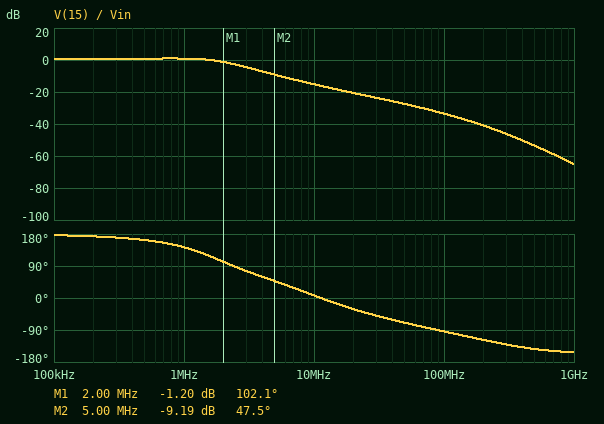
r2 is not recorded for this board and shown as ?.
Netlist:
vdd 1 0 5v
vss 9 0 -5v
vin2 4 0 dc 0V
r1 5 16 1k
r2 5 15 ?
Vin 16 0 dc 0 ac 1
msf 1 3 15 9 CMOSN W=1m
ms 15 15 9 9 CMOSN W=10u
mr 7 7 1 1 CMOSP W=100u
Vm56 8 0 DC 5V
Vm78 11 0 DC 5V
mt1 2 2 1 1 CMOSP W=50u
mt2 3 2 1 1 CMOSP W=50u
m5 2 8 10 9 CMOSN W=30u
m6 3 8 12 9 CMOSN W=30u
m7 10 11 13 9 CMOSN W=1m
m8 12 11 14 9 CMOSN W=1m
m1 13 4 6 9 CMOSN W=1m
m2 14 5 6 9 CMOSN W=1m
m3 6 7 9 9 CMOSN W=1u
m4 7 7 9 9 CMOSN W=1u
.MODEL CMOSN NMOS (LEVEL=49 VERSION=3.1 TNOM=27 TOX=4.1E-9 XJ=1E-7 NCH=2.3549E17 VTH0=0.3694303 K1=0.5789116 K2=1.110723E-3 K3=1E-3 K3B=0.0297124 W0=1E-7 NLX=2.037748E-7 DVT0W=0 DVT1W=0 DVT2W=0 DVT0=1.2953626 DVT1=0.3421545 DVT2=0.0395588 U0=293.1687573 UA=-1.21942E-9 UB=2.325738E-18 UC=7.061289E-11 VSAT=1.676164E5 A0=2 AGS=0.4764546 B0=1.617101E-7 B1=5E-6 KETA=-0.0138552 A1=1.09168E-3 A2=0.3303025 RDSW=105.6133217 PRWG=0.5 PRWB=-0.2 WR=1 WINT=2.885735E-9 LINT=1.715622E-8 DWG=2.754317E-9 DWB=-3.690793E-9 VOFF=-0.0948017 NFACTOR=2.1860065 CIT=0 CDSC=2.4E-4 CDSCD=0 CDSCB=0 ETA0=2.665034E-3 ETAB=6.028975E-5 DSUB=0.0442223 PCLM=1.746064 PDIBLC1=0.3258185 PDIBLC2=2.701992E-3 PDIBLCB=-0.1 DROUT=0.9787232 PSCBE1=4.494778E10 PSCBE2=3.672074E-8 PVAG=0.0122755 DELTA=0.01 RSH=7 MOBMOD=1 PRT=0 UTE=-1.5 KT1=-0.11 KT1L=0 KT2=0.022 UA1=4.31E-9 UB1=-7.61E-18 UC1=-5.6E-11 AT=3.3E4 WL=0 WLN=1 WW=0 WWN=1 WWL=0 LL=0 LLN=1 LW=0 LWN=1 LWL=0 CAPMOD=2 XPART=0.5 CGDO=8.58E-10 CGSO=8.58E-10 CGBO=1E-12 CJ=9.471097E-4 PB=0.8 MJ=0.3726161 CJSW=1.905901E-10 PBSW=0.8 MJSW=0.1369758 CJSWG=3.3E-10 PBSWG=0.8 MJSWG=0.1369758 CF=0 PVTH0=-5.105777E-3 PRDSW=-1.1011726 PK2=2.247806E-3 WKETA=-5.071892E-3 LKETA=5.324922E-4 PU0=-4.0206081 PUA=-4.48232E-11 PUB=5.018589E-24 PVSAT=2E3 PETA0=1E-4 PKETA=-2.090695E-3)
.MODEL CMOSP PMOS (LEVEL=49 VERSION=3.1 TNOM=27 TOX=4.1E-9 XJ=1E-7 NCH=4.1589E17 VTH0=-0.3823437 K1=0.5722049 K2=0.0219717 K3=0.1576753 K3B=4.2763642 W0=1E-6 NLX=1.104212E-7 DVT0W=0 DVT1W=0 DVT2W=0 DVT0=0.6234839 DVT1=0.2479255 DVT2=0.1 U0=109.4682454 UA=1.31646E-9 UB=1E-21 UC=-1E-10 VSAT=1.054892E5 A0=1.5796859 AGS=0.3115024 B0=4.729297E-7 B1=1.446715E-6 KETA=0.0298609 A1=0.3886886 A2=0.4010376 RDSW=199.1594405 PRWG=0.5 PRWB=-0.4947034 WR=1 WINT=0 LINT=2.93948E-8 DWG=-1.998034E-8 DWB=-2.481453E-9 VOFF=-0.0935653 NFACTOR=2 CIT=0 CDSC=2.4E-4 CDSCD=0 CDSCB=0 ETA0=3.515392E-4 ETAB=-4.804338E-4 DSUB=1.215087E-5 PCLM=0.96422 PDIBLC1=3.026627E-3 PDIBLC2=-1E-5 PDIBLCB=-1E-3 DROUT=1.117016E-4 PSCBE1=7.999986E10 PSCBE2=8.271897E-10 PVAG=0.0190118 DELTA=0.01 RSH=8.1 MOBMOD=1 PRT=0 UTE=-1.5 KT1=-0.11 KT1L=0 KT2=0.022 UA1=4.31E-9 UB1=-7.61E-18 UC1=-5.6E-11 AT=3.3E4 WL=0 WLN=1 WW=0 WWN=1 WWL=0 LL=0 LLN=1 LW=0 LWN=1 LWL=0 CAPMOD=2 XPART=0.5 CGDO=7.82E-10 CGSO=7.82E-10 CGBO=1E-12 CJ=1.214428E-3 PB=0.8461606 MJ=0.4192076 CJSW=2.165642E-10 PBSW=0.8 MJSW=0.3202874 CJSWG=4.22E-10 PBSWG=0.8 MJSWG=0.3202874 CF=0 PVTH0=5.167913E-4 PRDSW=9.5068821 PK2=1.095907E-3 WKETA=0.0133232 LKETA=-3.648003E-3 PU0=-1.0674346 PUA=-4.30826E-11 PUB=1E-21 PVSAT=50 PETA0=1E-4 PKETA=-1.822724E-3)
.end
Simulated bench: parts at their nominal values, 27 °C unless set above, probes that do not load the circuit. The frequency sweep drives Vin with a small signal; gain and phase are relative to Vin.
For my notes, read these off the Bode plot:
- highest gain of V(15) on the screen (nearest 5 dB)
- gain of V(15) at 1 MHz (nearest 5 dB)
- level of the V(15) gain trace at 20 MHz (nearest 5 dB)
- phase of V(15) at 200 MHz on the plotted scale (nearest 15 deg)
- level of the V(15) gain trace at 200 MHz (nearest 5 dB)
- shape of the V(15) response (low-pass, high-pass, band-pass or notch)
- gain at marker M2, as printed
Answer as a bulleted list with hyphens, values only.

- 0 dB
- 0 dB
- -20 dB
- -120 deg
- -40 dB
- low-pass
- -9.19 dB
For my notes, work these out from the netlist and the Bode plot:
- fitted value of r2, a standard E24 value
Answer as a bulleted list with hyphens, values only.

- 1.1 kΩ
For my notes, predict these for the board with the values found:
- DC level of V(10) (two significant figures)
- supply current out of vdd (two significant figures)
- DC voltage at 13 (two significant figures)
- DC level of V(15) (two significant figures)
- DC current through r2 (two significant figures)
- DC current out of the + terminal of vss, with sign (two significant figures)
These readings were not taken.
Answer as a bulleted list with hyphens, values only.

- 3.1 V
- 3.0 mA
- 3.1 V
- 9.9 mV
- 4.7 µA
- -3.0 mA
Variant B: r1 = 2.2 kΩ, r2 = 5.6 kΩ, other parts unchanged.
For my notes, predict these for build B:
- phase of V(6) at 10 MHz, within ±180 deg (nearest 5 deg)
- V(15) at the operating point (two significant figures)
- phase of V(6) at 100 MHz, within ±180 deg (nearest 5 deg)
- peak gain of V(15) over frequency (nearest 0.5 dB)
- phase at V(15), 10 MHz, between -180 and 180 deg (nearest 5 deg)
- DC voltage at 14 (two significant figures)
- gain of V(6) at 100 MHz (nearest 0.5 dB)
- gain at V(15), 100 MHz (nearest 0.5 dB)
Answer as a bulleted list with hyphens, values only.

- -55 deg
- 17 mV
- -85 deg
- 8.0 dB
- -20 deg
- 1.5 V
- -32.5 dB
- -51.0 dB
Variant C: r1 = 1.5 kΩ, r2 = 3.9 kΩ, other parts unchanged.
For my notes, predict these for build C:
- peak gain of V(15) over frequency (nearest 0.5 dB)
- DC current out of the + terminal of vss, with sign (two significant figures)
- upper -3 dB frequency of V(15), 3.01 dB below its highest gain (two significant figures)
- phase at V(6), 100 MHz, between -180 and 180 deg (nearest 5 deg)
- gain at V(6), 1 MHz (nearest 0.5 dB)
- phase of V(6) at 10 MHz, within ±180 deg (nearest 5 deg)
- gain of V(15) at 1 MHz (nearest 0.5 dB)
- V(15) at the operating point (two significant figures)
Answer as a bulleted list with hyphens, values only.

- 8.0 dB
- -3.0 mA
- 1.4 MHz
- -80 deg
- -11.0 dB
- -45 deg
- 7.0 dB
- 17 mV
